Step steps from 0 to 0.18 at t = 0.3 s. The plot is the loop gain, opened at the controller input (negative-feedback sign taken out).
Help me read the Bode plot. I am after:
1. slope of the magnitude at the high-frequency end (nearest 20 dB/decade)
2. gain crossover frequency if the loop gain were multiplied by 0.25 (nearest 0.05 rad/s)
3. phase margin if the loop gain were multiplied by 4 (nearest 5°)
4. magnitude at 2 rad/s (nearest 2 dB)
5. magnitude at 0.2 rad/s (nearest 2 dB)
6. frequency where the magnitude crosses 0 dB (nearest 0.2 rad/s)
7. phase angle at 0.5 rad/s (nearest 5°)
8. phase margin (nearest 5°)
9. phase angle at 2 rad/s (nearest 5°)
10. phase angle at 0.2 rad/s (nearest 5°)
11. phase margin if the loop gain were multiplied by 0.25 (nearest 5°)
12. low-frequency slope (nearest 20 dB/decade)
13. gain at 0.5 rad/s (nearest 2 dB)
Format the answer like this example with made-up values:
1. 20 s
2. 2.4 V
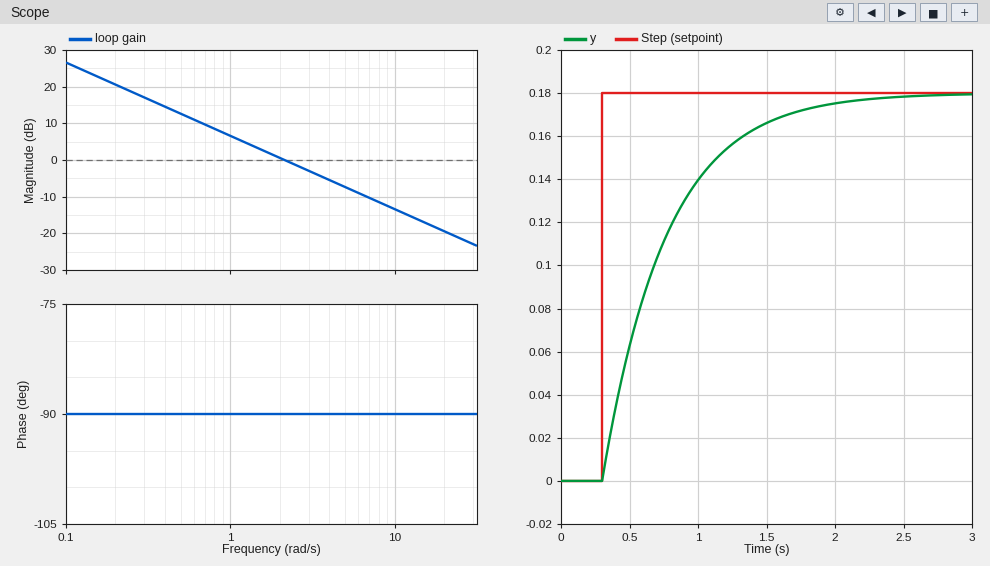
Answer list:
1. -20 dB/decade
2. 0.55 rad/s
3. 90°
4. 0 dB
5. 20 dB
6. 2.2 rad/s
7. -90°
8. 90°
9. -90°
10. -90°
11. 90°
12. -20 dB/decade
13. 12 dB
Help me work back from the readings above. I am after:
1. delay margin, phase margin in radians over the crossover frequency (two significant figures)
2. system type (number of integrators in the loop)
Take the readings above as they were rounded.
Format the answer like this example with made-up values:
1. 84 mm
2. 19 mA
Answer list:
1. 0.71 s
2. 1
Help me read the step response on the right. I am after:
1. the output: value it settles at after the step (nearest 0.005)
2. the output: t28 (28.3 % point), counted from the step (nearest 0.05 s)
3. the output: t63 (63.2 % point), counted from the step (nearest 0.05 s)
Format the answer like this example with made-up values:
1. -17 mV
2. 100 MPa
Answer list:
1. 0.180
2. 0.15 s
3. 0.45 s
